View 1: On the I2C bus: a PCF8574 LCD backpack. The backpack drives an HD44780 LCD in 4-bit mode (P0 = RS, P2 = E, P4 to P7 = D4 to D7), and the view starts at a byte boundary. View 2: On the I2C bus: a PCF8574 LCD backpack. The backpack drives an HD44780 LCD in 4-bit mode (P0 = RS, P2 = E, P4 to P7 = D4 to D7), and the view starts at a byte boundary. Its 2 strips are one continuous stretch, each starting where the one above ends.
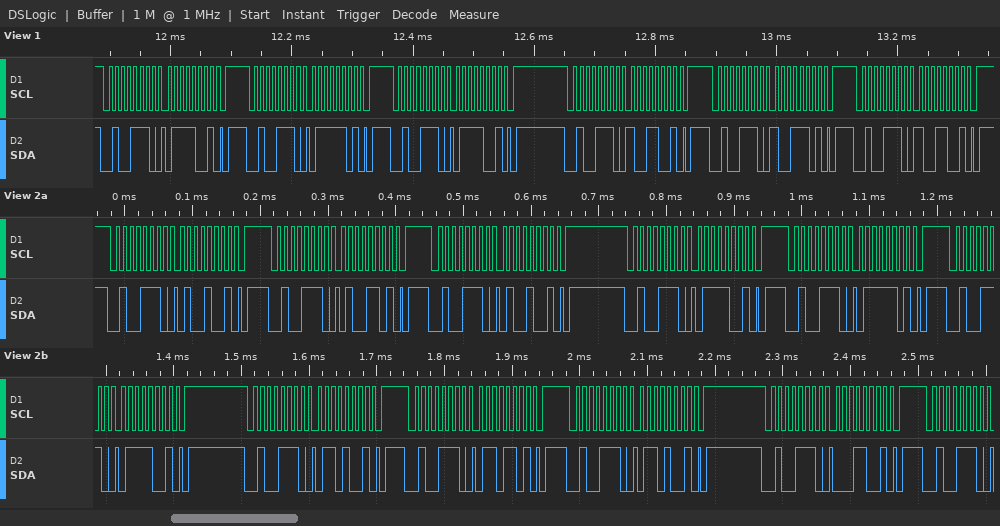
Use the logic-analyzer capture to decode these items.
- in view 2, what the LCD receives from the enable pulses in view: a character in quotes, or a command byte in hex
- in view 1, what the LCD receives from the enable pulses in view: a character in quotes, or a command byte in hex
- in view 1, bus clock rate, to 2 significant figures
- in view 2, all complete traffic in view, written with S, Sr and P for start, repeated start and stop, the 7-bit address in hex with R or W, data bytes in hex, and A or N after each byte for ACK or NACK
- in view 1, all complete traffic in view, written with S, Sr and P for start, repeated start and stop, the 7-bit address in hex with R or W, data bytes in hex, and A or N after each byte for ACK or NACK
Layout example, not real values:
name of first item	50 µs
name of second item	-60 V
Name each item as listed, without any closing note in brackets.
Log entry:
in view 2, what the LCD receives from the enable pulses in view: a character in quotes, or a command byte in hex	'G'
in view 1, what the LCD receives from the enable pulses in view: a character in quotes, or a command byte in hex	'y'
in view 1, bus clock rate, to 2 significant figures	100 kHz
in view 2, all complete traffic in view, written with S, Sr and P for start, repeated start and stop, the 7-bit address in hex with R or W, data bytes in hex, and A or N after each byte for ACK or NACK	S 27W A 49 A P S 27W A 4D A P S 27W A 49 A P S 27W A 79 A P S 27W A 7D A P S 27W A 79 A P S 27W A 69 A P S 27W A 6D A P S 27W A 69 A P S 27W A 19 A P S 27W A
in view 1, all complete traffic in view, written with S, Sr and P for start, repeated start and stop, the 7-bit address in hex with R or W, data bytes in hex, and A or N after each byte for ACK or NACK	S 27W A 79 A P S 27W A 7D A P S 27W A 79 A P S 27W A 99 A P S 27W A 9D A P S 27W A 99 A P
